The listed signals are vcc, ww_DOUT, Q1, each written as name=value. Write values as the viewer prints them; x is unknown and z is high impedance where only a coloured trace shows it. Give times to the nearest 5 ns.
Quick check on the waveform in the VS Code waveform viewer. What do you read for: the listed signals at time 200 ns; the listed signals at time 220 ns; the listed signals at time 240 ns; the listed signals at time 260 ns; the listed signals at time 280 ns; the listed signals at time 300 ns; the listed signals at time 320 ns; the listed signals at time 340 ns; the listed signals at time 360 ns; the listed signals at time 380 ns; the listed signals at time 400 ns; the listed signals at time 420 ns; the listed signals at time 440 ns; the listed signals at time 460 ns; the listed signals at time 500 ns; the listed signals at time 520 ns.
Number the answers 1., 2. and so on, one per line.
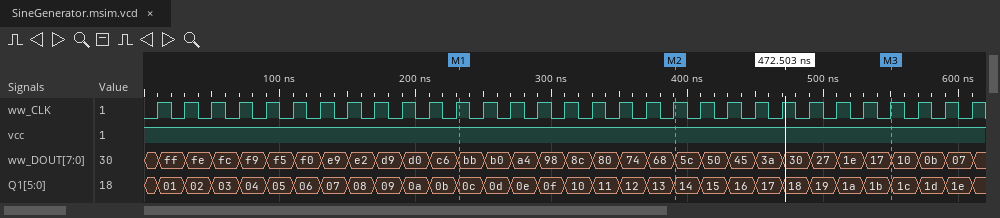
1. vcc=1, ww_DOUT=d0, Q1=0a
2. vcc=1, ww_DOUT=c6, Q1=0b
3. vcc=1, ww_DOUT=bb, Q1=0c
4. vcc=1, ww_DOUT=b0, Q1=0d
5. vcc=1, ww_DOUT=a4, Q1=0e
6. vcc=1, ww_DOUT=98, Q1=0f
7. vcc=1, ww_DOUT=8c, Q1=10
8. vcc=1, ww_DOUT=80, Q1=11
9. vcc=1, ww_DOUT=74, Q1=12
10. vcc=1, ww_DOUT=68, Q1=13
11. vcc=1, ww_DOUT=5c, Q1=14
12. vcc=1, ww_DOUT=50, Q1=15
13. vcc=1, ww_DOUT=45, Q1=16
14. vcc=1, ww_DOUT=3a, Q1=17
15. vcc=1, ww_DOUT=27, Q1=19
16. vcc=1, ww_DOUT=1e, Q1=1a
